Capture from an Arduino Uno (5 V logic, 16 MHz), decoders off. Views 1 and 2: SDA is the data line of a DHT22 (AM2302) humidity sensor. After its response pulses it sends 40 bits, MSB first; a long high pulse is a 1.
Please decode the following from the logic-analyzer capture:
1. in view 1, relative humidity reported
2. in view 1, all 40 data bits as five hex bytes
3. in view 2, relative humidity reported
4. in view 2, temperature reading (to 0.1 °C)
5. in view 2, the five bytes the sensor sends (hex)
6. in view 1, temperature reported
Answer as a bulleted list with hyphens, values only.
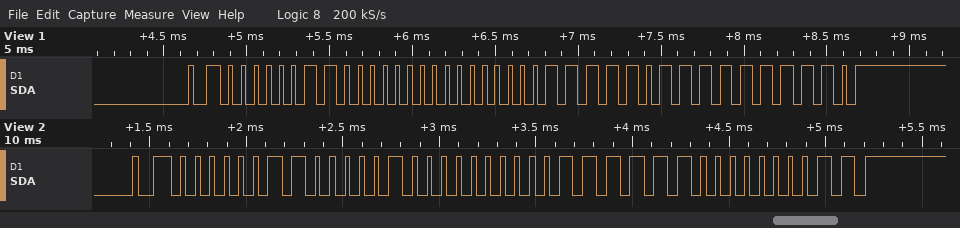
- 76.8 %
- 03 00 00 FB FE
- 77.2 %
- 25.2 °C
- 03 04 00 FC 03
- 25.1 °C
